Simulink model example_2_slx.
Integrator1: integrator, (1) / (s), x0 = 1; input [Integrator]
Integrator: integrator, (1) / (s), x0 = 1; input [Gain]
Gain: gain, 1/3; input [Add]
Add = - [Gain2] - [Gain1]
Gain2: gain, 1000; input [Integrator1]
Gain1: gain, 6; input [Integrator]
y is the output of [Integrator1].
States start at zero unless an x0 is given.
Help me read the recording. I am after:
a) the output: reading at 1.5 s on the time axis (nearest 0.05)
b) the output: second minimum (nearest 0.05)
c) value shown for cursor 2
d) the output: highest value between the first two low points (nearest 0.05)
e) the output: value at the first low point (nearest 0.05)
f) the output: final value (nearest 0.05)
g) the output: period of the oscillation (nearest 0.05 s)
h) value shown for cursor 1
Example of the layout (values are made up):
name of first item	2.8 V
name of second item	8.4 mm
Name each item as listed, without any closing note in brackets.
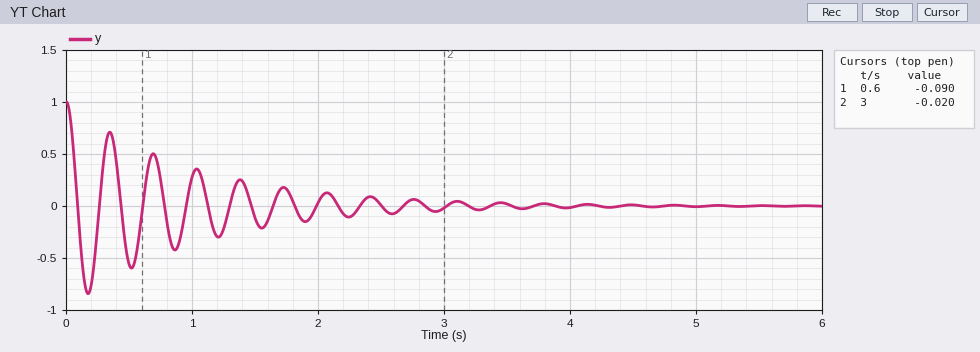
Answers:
the output: reading at 1.5 s on the time axis	-0.10
the output: second minimum	-0.60
value shown for cursor 2	-0.020
the output: highest value between the first two low points	0.70
the output: value at the first low point	-0.85
the output: final value	0.00
the output: period of the oscillation	0.35 s
value shown for cursor 1	-0.090
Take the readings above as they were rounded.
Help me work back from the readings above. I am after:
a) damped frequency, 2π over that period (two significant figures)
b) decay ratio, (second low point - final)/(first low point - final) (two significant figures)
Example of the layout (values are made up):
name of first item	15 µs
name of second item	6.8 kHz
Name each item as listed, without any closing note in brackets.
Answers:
damped frequency, 2π over that period	18 rad/s
decay ratio, (second low point - final)/(first low point - final)	0.71
